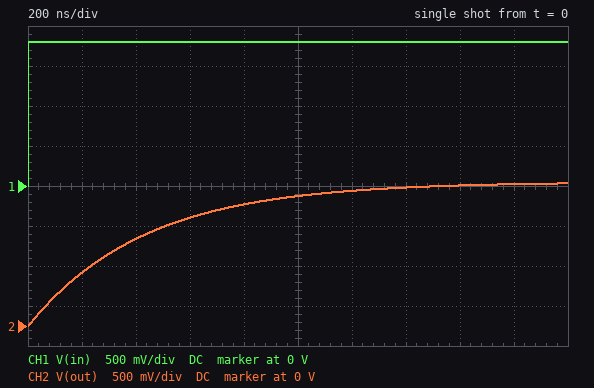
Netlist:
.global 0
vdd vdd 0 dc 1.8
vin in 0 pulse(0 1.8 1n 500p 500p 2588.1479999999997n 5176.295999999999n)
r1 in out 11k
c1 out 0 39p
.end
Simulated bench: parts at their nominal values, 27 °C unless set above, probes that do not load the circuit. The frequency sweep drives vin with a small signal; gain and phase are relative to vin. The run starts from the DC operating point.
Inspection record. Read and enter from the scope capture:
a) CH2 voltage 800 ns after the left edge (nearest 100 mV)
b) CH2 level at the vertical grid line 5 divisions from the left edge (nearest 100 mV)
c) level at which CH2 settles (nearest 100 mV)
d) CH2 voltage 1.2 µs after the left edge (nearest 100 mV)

1.5 V
1.6 V
1.8 V
1.7 V
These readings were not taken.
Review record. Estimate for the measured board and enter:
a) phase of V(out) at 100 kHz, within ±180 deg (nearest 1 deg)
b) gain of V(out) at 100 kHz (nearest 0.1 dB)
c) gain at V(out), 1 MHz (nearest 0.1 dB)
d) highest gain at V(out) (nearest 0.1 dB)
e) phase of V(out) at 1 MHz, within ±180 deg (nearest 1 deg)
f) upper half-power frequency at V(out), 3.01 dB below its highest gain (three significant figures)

-15 deg
-0.3 dB
-9.2 dB
0 dB
-70 deg
371 kHz
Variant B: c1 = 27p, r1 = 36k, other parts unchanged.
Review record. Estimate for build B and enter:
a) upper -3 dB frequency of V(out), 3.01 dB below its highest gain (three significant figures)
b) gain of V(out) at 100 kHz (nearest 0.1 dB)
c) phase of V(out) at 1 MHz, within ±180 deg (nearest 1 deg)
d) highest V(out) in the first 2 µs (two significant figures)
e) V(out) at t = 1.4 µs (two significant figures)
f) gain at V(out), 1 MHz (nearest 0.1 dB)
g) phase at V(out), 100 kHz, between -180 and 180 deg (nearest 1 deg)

164 kHz
-1.4 dB
-81 deg
1.6 V
1.4 V
-15.8 dB
-31 deg
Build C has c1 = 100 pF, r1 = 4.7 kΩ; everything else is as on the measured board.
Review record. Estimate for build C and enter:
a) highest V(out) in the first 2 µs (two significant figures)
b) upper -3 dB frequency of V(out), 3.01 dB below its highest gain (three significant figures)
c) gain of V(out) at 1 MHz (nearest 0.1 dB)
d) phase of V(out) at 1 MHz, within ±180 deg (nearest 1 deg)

1.8 V
339 kHz
-9.9 dB
-71 deg
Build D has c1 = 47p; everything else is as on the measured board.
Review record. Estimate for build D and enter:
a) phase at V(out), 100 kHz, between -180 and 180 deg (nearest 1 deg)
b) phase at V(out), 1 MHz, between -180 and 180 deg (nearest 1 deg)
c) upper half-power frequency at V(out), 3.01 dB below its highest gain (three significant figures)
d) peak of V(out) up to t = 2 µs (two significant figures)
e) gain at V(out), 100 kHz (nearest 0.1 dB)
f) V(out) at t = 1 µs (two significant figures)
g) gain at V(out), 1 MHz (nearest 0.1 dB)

-18 deg
-73 deg
308 kHz
1.8 V
-0.4 dB
1.5 V
-10.6 dB
